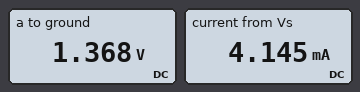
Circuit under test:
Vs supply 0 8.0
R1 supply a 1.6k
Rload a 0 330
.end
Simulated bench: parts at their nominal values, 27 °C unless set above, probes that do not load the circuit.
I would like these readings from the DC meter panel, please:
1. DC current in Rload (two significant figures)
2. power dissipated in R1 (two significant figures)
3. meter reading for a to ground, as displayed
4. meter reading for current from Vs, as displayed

4.1 mA
27 mW
1.368 V
4.145 mA
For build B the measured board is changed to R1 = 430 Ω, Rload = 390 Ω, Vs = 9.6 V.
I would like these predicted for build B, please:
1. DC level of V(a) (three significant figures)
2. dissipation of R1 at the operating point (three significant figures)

4.57 V
58.9 mW
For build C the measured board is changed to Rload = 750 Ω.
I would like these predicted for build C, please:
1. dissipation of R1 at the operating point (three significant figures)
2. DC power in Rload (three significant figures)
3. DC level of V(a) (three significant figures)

18.5 mW
8.69 mW
2.55 V
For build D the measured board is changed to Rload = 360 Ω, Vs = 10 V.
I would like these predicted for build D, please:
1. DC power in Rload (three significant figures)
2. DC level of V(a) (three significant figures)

9.37 mW
1.84 V
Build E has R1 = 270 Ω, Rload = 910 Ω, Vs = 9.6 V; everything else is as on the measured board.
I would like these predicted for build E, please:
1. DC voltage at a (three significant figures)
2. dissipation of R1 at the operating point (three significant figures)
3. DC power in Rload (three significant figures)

7.40 V
17.9 mW
60.2 mW
